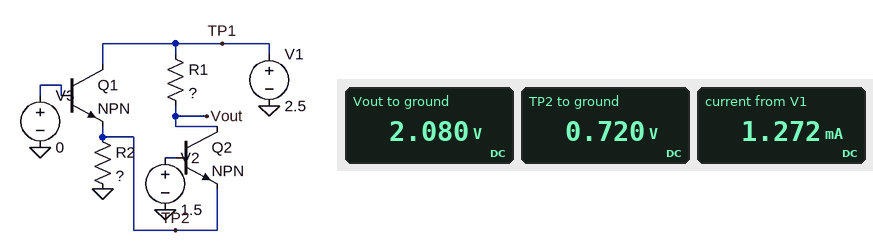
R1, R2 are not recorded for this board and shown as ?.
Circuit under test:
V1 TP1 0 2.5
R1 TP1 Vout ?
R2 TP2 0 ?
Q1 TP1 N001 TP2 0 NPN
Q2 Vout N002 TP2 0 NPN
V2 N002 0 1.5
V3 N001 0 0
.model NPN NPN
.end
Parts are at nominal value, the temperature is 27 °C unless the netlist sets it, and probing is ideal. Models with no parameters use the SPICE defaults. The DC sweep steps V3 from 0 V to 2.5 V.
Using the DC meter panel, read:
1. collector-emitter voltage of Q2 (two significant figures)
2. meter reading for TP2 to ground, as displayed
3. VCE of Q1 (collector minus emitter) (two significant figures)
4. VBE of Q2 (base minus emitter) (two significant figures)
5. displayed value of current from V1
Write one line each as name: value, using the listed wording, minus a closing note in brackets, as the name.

collector-emitter voltage of Q2: 1.4 V
meter reading for TP2 to ground, as displayed: 0.720 V
VCE of Q1 (collector minus emitter): 1.8 V
VBE of Q2 (base minus emitter): 780 mV
displayed value of current from V1: 1.272 mA
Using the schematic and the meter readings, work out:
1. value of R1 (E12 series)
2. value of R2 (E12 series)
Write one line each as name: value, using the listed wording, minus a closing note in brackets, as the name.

value of R1: 330 Ω
value of R2: 560 Ω
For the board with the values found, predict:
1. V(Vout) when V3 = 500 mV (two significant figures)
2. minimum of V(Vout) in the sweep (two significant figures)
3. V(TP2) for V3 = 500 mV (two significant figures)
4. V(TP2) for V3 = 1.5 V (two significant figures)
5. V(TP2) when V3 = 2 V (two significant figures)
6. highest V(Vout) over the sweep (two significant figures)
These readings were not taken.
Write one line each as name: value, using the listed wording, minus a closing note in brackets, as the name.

V(Vout) when V3 = 500 mV: 2.1 V
minimum of V(Vout) in the sweep: 2.1 V
V(TP2) for V3 = 500 mV: 720 mV
V(TP2) for V3 = 1.5 V: 740 mV
V(TP2) when V3 = 2 V: 1.2 V
highest V(Vout) over the sweep: 2.5 V
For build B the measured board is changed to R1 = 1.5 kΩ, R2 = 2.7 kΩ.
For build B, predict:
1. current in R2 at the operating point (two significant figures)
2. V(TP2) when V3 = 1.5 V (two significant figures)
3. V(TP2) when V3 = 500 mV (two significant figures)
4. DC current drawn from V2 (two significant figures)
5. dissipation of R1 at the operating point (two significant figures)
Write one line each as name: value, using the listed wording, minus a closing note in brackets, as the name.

current in R2 at the operating point: 280 µA
V(TP2) when V3 = 1.5 V: 780 mV
V(TP2) when V3 = 500 mV: 760 mV
DC current drawn from V2: 2.8 µA
dissipation of R1 at the operating point: 120 µW
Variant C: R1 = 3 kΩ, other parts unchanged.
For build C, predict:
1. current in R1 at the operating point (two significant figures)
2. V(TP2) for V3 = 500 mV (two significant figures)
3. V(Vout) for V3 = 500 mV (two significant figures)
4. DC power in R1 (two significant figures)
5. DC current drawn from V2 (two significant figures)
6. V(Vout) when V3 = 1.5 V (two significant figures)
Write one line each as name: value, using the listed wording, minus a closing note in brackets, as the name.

current in R1 at the operating point: 590 µA
V(TP2) for V3 = 500 mV: 710 mV
V(Vout) for V3 = 500 mV: 740 mV
DC power in R1: 1.0 mW
DC current drawn from V2: 680 µA
V(Vout) when V3 = 1.5 V: 800 mV
